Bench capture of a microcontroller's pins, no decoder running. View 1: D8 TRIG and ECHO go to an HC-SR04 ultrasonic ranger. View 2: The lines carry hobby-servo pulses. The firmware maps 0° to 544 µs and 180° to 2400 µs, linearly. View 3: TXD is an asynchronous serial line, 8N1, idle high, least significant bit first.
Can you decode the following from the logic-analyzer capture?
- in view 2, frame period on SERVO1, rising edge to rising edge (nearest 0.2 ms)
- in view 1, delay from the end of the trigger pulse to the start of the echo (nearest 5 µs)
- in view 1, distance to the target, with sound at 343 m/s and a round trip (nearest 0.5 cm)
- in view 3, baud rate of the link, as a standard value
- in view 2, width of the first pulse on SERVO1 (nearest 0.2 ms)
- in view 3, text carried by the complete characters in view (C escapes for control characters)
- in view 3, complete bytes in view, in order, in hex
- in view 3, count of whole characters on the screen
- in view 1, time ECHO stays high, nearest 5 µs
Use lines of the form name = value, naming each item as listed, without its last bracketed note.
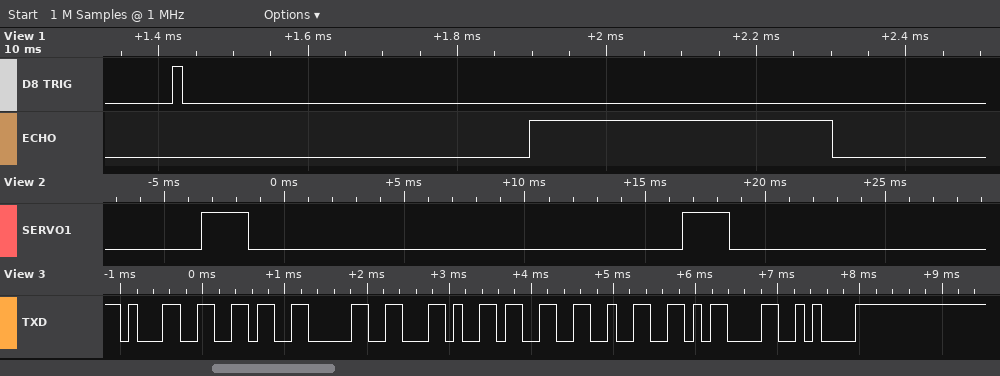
in view 2, frame period on SERVO1, rising edge to rising edge = 20.0 ms
in view 1, delay from the end of the trigger pulse to the start of the echo = 465 µs
in view 1, distance to the target, with sound at 343 m/s and a round trip = 7 cm
in view 3, baud rate of the link, as a standard value = 9600 baud
in view 2, width of the first pulse on SERVO1 = 2.0 ms
in view 3, text carried by the complete characters in view = "160,32\r\n"
in view 3, complete bytes in view, in order, in hex = 31 36 30 2C 33 32 0D 0A
in view 3, count of whole characters on the screen = 8
in view 1, time ECHO stays high, nearest 5 µs = 405 µs
